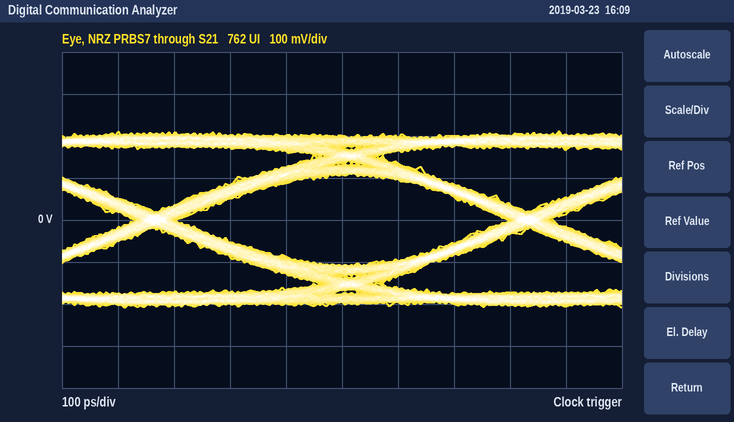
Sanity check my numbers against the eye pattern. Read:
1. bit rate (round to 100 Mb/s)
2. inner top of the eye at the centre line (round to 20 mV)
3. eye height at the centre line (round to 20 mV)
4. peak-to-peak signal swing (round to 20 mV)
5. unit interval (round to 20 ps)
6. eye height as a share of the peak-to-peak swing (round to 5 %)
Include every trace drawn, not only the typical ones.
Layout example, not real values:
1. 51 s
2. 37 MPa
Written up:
1. 1.5 Gb/s
2. 100 mV
3. 220 mV
4. 420 mV
5. 660 ps
6. 50 %
